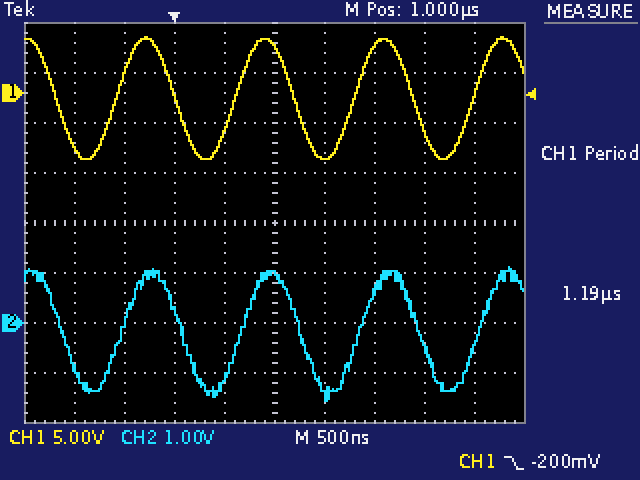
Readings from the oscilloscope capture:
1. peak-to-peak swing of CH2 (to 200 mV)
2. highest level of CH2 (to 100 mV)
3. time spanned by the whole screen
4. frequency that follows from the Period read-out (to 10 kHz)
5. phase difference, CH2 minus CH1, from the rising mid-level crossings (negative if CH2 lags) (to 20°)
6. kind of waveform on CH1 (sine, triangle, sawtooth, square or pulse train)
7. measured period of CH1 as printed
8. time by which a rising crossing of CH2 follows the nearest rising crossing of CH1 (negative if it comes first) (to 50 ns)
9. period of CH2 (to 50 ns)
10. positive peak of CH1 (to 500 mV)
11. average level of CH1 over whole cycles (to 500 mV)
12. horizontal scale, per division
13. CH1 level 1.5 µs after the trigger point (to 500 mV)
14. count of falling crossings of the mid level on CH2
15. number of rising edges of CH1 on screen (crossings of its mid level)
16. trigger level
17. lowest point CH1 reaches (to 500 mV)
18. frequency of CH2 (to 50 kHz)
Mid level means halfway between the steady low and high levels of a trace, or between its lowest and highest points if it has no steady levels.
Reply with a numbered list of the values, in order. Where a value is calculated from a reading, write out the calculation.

1. 2.6 V
2. 1.1 V
3. 5 µs
4. 1 / 1.19 µs ≈ 840 kHz
5. −360° × (+50 ns) / 1.20 µs ≈ -15.0°, so -20° to the nearest 20°
6. sine
7. 1.19 µs
8. +50 ns
9. 1.20 µs
10. 5.5 V
11. (5.5 V + (-6.5 V)) / 2 ≈ -500 mV
12. 500 ns
13. -6.5 V
14. 4
15. 4
16. -200 mV
17. -6.5 V
18. 1 / 1.20 µs ≈ 833 kHz, so 850 kHz to the nearest 50 kHz
